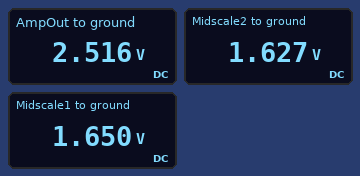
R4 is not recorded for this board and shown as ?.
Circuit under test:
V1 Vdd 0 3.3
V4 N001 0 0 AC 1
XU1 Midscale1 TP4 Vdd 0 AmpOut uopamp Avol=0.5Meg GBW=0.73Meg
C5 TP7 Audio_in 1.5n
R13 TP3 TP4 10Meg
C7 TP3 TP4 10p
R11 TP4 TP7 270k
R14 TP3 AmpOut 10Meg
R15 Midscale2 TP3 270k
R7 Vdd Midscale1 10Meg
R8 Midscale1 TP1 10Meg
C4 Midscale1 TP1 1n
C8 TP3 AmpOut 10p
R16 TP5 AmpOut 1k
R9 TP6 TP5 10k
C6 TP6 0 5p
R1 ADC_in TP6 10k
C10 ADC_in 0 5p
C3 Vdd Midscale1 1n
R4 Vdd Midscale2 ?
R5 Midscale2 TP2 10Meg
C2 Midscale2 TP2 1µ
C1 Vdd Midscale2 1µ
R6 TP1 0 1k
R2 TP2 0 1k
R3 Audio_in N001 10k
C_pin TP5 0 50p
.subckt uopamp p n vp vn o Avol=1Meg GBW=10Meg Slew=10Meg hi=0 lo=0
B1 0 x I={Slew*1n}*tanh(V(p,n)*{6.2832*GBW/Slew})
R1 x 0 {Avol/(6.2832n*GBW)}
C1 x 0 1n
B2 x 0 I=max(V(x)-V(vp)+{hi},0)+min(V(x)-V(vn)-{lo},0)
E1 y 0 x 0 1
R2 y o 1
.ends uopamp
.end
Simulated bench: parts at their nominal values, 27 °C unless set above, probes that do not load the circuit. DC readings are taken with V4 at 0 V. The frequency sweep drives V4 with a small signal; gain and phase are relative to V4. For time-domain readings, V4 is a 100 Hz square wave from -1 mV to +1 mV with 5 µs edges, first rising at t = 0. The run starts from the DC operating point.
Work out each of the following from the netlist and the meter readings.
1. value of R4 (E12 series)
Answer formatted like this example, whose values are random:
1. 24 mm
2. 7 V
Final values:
1. 22 MΩ
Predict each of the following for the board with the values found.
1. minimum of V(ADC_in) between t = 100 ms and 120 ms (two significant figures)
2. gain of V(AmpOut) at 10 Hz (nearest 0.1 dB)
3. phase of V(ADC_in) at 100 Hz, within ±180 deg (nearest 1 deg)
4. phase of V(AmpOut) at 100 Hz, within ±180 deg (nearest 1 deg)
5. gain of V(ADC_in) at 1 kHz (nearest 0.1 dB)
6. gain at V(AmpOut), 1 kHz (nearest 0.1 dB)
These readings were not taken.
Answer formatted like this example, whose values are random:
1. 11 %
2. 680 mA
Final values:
1. 1.3 V
2. 31.3 dB
3. -113 deg
4. -113 deg
5. 52.9 dB
6. 52.9 dB
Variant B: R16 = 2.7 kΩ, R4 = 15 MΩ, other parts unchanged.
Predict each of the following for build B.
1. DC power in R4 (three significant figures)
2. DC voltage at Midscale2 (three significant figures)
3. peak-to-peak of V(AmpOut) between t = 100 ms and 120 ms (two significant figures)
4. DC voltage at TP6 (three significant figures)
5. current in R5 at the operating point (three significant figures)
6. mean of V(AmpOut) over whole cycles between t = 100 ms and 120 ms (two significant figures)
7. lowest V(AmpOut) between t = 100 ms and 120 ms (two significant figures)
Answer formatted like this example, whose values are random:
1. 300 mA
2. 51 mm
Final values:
1. 185 nW
2. 1.64 V
3. 2.3 V
4. 2.18 V
5. 164 nA
6. 2.2 V
7. 970 mV
